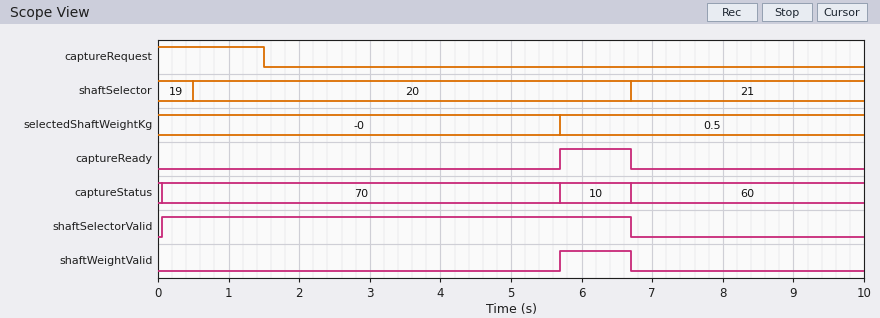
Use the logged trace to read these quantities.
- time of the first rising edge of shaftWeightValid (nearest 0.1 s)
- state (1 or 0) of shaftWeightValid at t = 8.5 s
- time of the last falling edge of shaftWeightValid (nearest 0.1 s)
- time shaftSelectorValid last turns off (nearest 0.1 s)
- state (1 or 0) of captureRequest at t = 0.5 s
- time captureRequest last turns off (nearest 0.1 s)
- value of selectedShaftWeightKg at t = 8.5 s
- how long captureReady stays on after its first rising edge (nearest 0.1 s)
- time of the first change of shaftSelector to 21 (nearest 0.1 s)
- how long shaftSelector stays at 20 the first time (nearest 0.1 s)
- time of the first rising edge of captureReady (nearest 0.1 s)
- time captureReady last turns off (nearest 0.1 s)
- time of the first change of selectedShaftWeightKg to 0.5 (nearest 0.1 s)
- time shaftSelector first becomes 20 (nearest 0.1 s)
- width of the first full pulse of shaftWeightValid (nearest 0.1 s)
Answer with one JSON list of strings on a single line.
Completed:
["5.7 s", "0", "6.7 s", "6.7 s", "1", "1.5 s", "0.5", "1.0 s", "6.7 s", "6.2 s", "5.7 s", "6.7 s", "5.7 s", "0.5 s", "1.0 s"]
